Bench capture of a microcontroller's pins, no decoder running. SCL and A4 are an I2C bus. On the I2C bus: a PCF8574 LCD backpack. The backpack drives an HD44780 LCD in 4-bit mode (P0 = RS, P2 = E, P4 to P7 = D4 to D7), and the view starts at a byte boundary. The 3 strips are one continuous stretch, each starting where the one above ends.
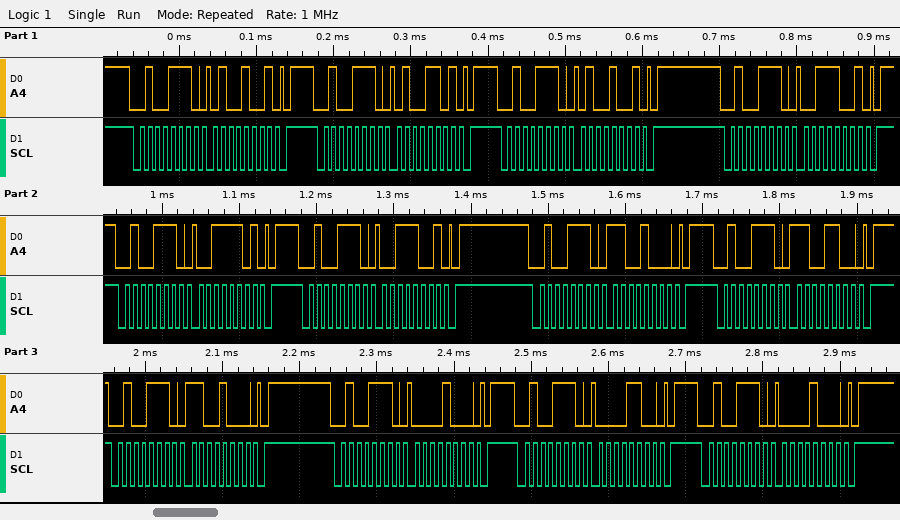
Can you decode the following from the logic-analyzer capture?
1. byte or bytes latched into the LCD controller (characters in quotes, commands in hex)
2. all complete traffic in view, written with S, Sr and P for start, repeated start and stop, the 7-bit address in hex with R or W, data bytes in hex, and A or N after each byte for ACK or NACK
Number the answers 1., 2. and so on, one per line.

1. 'C' 0xC0
2. S 27W A 49 A P S 27W A 4D A P S 27W A 49 A P S 27W A 39 A P S 27W A 3D A P S 27W A 39 A P S 27W A C8 A P S 27W A CC A P S 27W A C8 A P S 27W A 08 A P S 27W A 0C A P S 27W A 08 A P
